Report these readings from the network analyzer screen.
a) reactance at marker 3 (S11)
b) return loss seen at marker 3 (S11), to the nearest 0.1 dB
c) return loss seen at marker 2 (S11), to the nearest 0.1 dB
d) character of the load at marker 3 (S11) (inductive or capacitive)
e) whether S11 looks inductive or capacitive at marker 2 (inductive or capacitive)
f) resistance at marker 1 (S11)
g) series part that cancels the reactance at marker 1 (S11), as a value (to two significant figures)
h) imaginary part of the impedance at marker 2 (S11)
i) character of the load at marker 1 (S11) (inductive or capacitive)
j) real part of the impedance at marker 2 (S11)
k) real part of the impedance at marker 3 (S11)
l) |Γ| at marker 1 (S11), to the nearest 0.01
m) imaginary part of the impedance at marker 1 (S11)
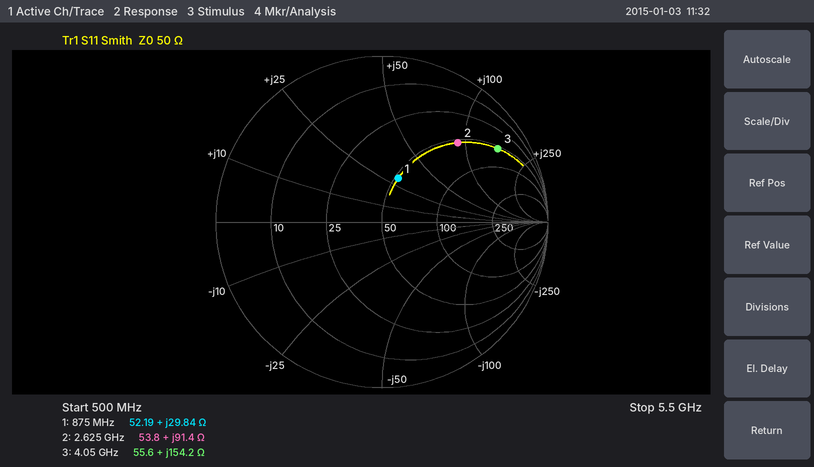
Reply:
+154.2 Ω
1.7 dB
3.6 dB
inductive
inductive
52.19 Ω
6.1 pF
+91.4 Ω
inductive
53.8 Ω
55.6 Ω
0.28
+29.84 Ω
